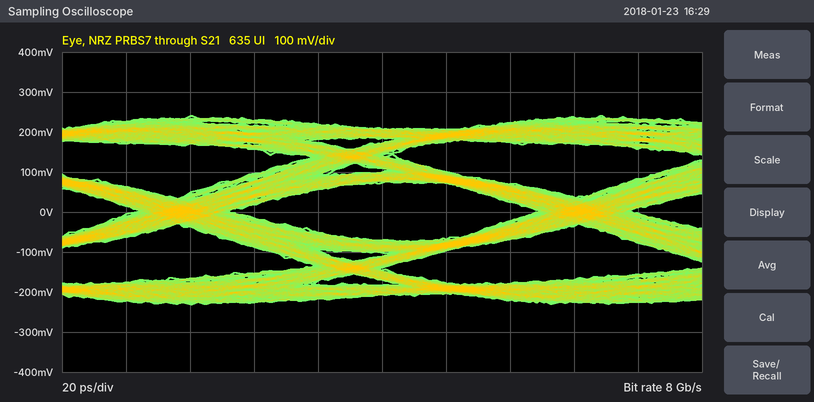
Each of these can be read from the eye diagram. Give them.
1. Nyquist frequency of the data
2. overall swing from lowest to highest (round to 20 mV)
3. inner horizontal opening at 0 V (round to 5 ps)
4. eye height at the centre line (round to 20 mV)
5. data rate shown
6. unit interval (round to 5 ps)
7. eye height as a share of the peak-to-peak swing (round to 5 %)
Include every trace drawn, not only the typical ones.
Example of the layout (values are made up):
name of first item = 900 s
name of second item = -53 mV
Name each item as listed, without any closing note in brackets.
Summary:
Nyquist frequency of the data = 4 GHz
overall swing from lowest to highest = 480 mV
inner horizontal opening at 0 V = 95 ps
eye height at the centre line = 140 mV
data rate shown = 8 Gb/s
unit interval = 125 ps
eye height as a share of the peak-to-peak swing = 30 %
